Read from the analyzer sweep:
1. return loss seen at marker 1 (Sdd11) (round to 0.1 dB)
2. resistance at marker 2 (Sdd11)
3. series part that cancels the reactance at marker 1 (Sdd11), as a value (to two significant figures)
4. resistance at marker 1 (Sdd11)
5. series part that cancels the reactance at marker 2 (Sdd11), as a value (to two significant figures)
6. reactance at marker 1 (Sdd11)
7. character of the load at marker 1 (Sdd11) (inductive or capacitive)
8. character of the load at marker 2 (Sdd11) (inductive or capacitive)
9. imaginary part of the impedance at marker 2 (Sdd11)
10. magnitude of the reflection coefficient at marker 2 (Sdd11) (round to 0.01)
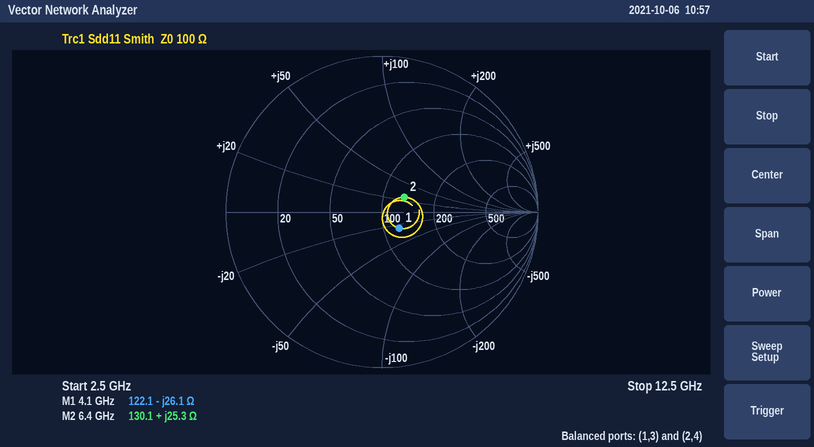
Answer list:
16.3 dB
130.1 Ω
1.0 nH
122.1 Ω
980 fF
-26.1 Ω
capacitive
inductive
+25.3 Ω
0.17
